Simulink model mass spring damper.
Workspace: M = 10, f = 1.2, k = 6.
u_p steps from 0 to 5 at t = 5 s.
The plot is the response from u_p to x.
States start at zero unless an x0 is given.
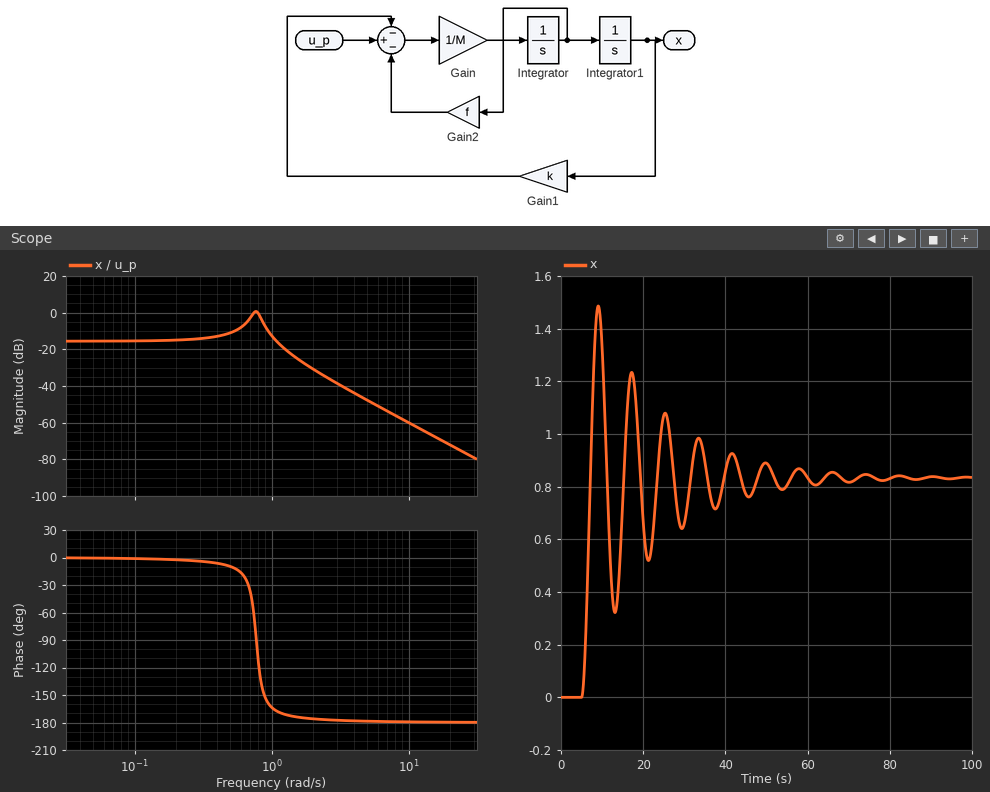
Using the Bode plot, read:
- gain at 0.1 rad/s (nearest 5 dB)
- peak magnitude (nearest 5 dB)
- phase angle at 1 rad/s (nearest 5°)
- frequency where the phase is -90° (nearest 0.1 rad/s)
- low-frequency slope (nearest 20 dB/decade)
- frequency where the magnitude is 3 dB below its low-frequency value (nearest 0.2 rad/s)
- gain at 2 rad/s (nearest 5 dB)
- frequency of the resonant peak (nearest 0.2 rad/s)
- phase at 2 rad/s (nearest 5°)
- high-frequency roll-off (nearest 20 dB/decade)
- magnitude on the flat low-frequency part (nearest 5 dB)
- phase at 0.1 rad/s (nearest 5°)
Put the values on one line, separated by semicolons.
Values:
-15 dB; 0 dB; -165°; 0.8 rad/s; 0 dB/decade; 1.2 rad/s; -30 dB; 0.8 rad/s; -175°; -40 dB/decade; -15 dB; 0°
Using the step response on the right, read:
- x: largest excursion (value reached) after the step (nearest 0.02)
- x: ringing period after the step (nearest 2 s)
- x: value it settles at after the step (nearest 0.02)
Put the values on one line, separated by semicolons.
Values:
1.48; 8 s; 0.84
